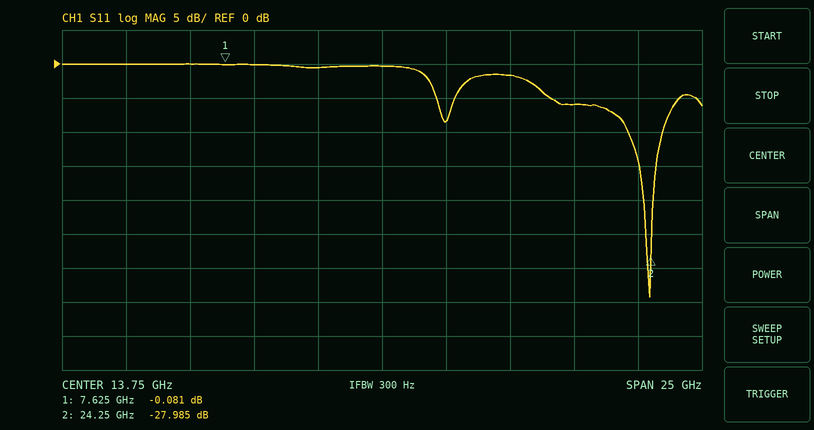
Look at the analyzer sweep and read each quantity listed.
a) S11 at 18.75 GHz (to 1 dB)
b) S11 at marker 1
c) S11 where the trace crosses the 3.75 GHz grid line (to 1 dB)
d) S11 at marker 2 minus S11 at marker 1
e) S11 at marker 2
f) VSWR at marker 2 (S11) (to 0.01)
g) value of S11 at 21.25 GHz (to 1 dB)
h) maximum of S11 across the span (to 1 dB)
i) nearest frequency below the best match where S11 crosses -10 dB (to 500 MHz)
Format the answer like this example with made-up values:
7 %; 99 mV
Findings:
-2 dB; -0.081 dB; 0 dB; -27.904 dB; -27.985 dB; 1.08; -6 dB; 0 dB; 23.5 GHz
